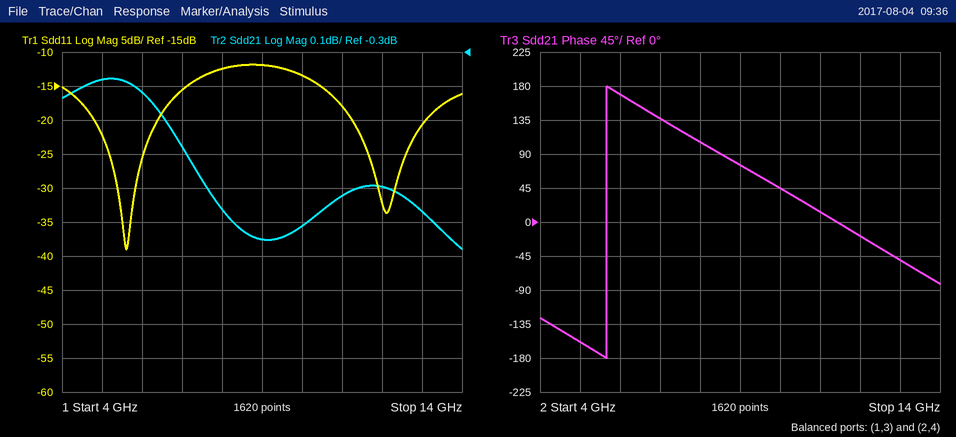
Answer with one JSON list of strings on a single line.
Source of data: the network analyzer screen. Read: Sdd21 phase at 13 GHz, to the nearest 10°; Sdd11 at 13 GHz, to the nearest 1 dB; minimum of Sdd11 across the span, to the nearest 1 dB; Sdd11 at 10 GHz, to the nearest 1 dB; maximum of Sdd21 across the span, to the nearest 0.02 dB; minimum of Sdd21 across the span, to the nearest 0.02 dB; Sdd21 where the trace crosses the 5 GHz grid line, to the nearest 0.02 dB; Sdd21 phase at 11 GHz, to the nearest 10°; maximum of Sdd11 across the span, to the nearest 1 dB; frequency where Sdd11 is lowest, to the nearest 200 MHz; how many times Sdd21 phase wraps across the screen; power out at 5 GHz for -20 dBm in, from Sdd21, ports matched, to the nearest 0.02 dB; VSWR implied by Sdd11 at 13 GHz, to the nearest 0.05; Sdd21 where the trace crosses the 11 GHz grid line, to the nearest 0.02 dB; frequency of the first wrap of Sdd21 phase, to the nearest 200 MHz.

["-50°", "-21 dB", "-39 dB", "-13 dB", "-0.38 dB", "-0.88 dB", "-0.38 dB", "10°", "-12 dB", "5.6 GHz", "1", "-20.38 dBm", "1.20", "-0.72 dB", "5.6 GHz"]
